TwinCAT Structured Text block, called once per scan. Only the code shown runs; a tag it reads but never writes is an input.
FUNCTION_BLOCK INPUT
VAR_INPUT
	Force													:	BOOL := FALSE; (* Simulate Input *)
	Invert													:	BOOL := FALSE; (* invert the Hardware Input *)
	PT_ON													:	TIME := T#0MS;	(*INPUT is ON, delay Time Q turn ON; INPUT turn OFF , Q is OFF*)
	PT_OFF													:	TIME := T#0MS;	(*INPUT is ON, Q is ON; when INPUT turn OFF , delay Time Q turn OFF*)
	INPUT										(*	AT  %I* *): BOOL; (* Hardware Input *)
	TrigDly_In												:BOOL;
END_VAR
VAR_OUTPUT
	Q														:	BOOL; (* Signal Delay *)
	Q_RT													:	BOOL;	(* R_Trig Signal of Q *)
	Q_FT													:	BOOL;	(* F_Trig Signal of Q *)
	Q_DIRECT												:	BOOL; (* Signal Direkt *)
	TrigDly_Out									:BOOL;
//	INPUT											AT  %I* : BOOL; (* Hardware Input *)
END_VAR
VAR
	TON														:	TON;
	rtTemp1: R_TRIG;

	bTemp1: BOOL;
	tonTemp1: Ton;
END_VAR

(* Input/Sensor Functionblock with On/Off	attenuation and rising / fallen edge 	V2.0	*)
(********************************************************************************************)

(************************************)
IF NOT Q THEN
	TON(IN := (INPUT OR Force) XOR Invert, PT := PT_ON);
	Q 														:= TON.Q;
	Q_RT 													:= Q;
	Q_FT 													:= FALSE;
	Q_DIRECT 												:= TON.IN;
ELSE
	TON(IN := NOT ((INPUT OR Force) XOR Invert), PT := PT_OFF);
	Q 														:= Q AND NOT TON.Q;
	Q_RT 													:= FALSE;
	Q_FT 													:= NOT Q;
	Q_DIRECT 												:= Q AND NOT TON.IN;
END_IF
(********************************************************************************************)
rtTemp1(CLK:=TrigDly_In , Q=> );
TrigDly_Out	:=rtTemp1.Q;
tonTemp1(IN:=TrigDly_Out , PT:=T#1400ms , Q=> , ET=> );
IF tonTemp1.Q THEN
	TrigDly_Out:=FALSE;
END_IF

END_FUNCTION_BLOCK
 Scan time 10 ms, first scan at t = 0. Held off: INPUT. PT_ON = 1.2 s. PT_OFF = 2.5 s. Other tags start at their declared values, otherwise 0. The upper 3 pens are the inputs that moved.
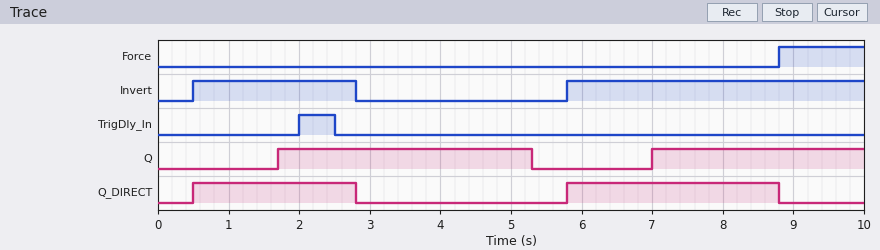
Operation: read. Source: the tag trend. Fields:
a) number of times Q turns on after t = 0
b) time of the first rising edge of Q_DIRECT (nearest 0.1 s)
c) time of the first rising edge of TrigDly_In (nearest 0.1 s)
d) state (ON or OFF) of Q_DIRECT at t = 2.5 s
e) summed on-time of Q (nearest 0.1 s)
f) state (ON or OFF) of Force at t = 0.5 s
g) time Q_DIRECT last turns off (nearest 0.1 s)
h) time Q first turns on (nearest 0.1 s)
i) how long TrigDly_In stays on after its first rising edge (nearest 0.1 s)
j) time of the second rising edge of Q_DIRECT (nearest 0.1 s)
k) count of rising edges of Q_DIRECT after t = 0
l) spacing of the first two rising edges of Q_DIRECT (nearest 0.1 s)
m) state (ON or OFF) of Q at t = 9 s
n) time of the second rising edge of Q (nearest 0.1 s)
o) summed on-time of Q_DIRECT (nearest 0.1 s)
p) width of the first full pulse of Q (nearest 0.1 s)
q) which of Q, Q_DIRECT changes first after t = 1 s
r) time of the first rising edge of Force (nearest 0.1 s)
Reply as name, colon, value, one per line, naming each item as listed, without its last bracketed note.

number of times Q turns on after t = 0: 2
time of the first rising edge of Q_DIRECT: 0.5 s
time of the first rising edge of TrigDly_In: 2.0 s
state (ON or OFF) of Q_DIRECT at t = 2.5 s: ON
summed on-time of Q: 6.6 s
state (ON or OFF) of Force at t = 0.5 s: OFF
time Q_DIRECT last turns off: 8.8 s
time Q first turns on: 1.7 s
how long TrigDly_In stays on after its first rising edge: 0.5 s
time of the second rising edge of Q_DIRECT: 5.8 s
count of rising edges of Q_DIRECT after t = 0: 2
spacing of the first two rising edges of Q_DIRECT: 5.3 s
state (ON or OFF) of Q at t = 9 s: ON
time of the second rising edge of Q: 7.0 s
summed on-time of Q_DIRECT: 5.3 s
width of the first full pulse of Q: 3.6 s
which of Q, Q_DIRECT changes first after t = 1 s: Q
time of the first rising edge of Force: 8.8 s
